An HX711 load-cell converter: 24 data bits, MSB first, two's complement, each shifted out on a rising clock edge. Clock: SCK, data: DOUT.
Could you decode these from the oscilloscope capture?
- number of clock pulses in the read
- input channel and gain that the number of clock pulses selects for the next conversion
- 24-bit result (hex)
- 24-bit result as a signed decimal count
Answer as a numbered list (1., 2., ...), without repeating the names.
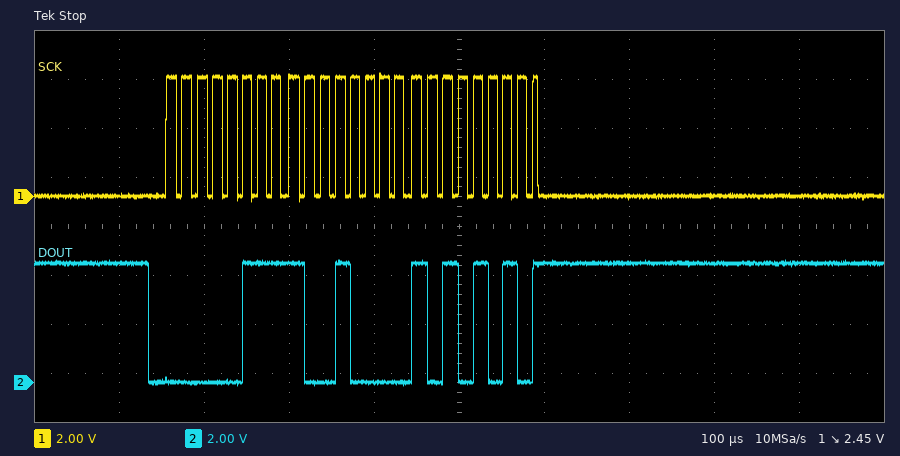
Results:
1. 25
2. channel A, gain 128
3. 0x0790AA
4. 495786
